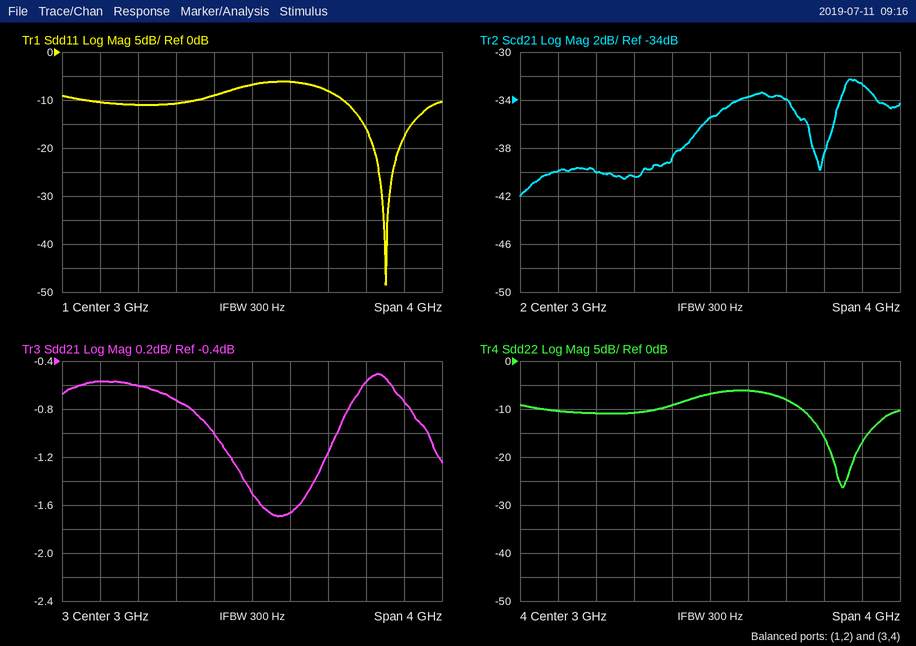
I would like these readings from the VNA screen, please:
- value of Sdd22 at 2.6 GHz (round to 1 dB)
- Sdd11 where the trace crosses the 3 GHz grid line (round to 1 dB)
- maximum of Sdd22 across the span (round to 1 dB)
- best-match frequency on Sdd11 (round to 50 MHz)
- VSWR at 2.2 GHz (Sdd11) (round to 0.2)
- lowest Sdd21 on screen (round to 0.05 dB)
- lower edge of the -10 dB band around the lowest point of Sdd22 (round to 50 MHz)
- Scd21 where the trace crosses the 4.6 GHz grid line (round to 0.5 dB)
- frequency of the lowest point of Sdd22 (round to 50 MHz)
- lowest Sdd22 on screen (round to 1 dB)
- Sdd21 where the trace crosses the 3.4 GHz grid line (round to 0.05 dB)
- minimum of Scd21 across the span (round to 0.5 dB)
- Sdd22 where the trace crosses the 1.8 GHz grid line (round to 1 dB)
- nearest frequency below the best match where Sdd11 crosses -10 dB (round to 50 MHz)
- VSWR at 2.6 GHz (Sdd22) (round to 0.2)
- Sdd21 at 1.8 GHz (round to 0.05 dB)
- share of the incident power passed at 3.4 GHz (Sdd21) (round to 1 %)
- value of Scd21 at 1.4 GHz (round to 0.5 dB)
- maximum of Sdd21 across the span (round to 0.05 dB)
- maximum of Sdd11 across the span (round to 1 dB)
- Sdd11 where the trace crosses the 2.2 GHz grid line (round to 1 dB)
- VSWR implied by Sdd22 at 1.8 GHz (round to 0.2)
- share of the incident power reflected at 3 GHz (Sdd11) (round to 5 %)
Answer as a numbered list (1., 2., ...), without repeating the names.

1. -9 dB
2. -7 dB
3. -6 dB
4. 4.40 GHz
5. 1.8
6. -1.70 dB
7. 3.95 GHz
8. -32.5 dB
9. 4.40 GHz
10. -26 dB
11. -1.65 dB
12. -42.0 dB
13. -11 dB
14. 3.95 GHz
15. 2.0
16. -0.60 dB
17. 68 %
18. -40.0 dB
19. -0.50 dB
20. -6 dB
21. -11 dB
22. 1.8
23. 20 %
